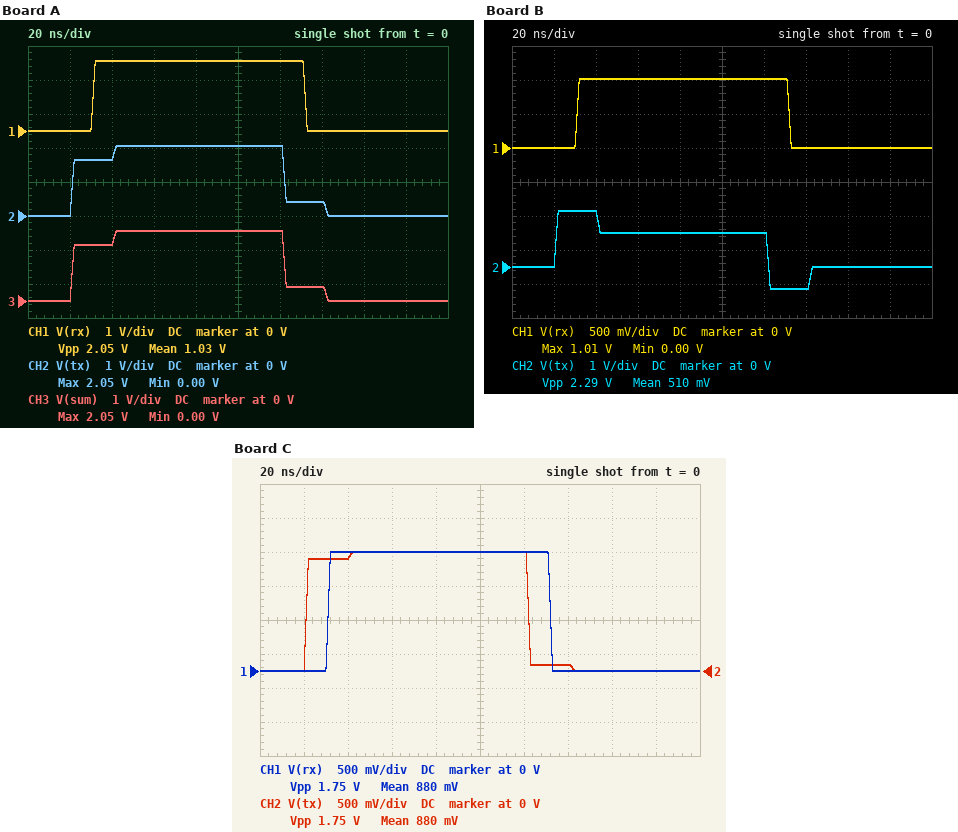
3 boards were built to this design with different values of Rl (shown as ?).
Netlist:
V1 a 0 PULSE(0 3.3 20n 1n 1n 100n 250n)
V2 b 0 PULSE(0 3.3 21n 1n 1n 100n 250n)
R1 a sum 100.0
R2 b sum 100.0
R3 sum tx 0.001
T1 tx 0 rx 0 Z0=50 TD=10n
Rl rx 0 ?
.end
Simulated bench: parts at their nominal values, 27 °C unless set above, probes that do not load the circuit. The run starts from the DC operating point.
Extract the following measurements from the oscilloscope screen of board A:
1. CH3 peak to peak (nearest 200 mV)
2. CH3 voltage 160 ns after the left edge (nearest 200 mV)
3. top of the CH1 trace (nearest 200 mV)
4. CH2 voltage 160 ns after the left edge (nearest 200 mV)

2.0 V
0 V
2.0 V
0 V
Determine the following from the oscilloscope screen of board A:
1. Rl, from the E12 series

82 Ω
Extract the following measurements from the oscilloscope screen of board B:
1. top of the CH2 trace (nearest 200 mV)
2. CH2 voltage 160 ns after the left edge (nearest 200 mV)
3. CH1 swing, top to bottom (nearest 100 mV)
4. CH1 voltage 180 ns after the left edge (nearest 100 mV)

1.6 V
0 V
1.0 V
0 V
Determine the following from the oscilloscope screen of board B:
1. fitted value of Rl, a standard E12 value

22 Ω
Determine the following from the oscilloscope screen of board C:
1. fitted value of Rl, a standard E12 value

56 Ω
